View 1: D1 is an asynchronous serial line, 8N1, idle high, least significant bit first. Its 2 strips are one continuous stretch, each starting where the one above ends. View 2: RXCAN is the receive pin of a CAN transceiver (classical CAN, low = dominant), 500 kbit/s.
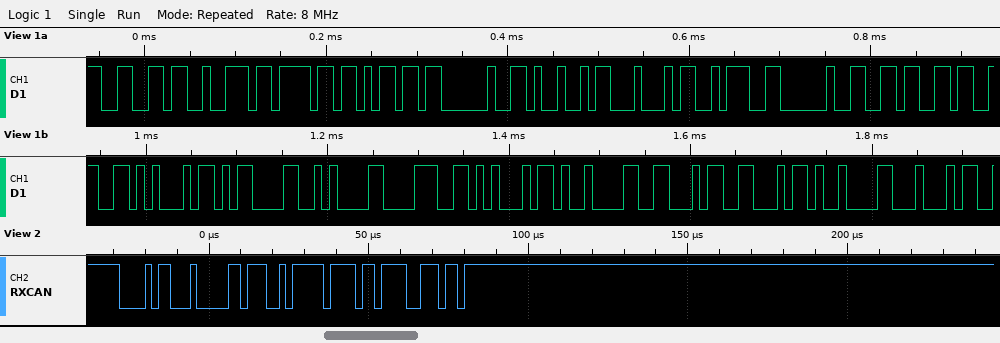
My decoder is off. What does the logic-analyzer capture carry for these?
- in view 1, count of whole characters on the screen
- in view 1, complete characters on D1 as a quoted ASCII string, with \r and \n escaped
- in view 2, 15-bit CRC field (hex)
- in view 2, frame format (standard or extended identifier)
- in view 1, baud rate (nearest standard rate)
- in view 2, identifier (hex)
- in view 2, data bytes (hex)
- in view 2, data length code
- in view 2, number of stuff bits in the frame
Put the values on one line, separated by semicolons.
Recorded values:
21; "from ID: 63E\r\n8E\tFF\tD"; 0x379D; standard; 115200 baud; 0x0B1; E5 FF; 2; 2
